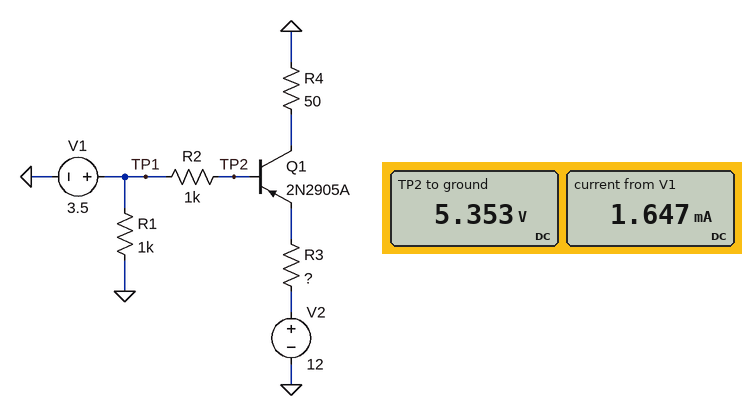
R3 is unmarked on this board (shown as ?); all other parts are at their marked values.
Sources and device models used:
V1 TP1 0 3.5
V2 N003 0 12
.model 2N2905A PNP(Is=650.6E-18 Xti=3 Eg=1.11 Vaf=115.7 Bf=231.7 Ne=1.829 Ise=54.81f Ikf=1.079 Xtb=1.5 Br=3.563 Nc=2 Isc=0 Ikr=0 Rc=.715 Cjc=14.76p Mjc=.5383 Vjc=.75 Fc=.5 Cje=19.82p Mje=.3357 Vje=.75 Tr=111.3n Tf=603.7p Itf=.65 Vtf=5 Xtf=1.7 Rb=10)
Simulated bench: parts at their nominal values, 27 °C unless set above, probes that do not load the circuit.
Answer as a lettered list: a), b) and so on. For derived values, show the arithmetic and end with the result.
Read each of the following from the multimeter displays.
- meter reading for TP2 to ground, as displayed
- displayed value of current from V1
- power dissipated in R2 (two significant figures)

a) 5.353 V
b) 1.647 mA
c) (5.353 V - 3.5 V)^2 / 1 kΩ = 3.4 mW
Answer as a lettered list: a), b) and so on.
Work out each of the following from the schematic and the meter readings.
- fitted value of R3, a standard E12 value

a) 47 Ω
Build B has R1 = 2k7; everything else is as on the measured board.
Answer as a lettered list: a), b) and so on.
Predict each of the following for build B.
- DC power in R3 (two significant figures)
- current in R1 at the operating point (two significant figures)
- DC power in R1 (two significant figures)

a) 710 mW
b) 1.3 mA
c) 4.5 mW
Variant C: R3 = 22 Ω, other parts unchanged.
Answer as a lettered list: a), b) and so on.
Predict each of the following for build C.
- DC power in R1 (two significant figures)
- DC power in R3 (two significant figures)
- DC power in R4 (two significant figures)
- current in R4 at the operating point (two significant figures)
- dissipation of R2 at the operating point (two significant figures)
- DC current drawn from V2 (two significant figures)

a) 12 mW
b) 610 mW
c) 1.3 W
d) 160 mA
e) 15 mW
f) 170 mA
